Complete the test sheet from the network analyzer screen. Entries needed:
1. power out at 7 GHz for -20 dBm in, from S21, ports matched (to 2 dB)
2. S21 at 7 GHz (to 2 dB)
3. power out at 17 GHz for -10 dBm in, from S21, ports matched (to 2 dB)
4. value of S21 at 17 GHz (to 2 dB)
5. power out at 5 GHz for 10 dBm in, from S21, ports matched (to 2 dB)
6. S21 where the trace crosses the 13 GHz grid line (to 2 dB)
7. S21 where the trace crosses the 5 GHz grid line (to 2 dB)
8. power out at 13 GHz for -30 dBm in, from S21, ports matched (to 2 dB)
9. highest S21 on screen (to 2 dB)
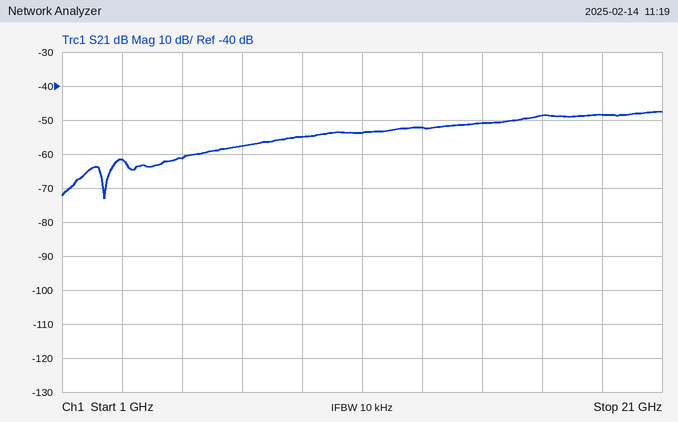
-78 dBm
-58 dB
-58 dBm
-48 dB
-52 dBm
-52 dB
-62 dB
-82 dBm
-48 dB
